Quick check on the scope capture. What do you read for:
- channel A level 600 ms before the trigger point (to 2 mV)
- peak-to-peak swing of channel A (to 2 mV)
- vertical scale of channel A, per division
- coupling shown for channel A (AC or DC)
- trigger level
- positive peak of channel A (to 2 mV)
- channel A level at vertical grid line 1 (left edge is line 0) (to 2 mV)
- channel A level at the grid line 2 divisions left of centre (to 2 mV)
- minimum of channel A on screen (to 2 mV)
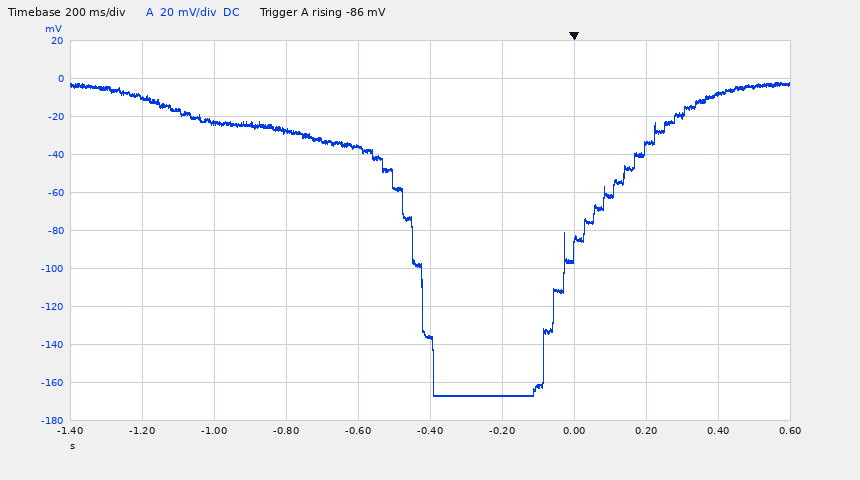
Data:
-36 mV
164 mV
20 mV
DC
-86 mV
-2 mV
-10 mV
-28 mV
-166 mV
